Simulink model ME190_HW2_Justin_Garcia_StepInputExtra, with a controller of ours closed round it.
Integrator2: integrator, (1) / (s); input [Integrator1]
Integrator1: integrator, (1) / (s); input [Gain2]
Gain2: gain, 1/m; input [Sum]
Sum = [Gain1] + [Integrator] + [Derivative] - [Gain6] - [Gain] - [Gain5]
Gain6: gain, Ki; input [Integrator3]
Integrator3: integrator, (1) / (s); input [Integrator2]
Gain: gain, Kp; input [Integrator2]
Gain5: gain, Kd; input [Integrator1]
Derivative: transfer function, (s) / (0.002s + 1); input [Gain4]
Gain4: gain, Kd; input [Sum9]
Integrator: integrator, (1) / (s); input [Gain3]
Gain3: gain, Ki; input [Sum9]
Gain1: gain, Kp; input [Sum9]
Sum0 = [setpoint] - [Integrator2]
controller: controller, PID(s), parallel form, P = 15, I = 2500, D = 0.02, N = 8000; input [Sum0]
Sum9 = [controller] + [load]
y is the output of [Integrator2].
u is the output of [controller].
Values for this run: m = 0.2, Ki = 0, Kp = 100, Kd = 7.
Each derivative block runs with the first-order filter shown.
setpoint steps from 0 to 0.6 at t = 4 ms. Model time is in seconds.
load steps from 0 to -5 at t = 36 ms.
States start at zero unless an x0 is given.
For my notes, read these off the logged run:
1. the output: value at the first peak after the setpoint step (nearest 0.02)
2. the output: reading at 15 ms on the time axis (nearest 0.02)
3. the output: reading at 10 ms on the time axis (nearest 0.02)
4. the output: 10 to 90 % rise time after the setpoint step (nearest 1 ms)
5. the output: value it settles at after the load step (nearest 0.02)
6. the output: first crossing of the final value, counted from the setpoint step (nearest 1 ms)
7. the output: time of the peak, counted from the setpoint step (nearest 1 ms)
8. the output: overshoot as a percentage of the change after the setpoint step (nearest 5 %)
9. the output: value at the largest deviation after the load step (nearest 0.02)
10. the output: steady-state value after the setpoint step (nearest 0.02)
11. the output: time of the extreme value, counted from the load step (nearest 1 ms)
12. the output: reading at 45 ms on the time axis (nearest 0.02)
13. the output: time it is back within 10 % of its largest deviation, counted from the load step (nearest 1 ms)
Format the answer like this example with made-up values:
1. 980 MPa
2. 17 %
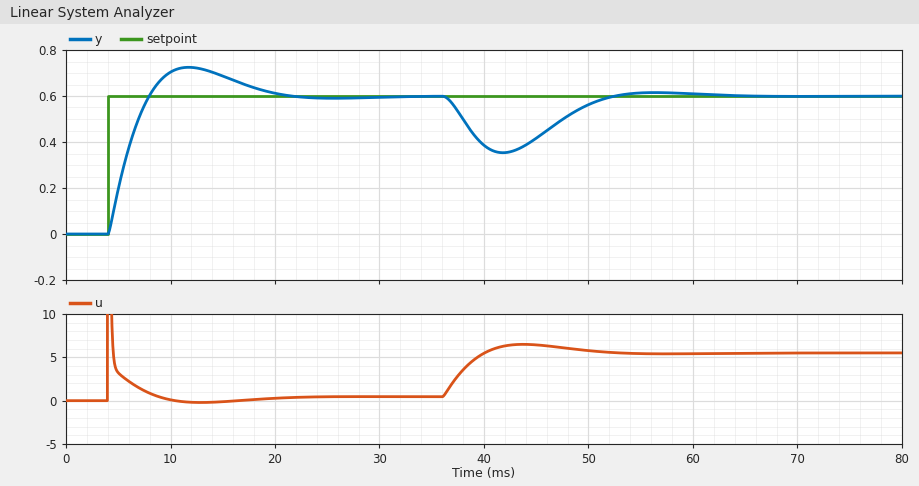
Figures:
1. 0.72
2. 0.68
3. 0.70
4. 3 ms
5. 0.60
6. 4 ms
7. 8 ms
8. 20 %
9. 0.36
10. 0.60
11. 6 ms
12. 0.42
13. 15 ms
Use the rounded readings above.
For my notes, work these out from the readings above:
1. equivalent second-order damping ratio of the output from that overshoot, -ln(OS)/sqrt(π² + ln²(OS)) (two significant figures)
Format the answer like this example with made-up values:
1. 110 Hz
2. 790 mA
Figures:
1. 0.46
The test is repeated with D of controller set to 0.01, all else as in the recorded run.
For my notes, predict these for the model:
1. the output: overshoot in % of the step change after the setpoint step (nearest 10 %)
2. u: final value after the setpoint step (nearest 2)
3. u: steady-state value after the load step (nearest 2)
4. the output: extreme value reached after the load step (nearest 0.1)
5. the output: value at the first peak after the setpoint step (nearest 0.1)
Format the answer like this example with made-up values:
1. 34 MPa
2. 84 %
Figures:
1. 30 %
2. 0
3. 6
4. 0.3
5. 0.8
